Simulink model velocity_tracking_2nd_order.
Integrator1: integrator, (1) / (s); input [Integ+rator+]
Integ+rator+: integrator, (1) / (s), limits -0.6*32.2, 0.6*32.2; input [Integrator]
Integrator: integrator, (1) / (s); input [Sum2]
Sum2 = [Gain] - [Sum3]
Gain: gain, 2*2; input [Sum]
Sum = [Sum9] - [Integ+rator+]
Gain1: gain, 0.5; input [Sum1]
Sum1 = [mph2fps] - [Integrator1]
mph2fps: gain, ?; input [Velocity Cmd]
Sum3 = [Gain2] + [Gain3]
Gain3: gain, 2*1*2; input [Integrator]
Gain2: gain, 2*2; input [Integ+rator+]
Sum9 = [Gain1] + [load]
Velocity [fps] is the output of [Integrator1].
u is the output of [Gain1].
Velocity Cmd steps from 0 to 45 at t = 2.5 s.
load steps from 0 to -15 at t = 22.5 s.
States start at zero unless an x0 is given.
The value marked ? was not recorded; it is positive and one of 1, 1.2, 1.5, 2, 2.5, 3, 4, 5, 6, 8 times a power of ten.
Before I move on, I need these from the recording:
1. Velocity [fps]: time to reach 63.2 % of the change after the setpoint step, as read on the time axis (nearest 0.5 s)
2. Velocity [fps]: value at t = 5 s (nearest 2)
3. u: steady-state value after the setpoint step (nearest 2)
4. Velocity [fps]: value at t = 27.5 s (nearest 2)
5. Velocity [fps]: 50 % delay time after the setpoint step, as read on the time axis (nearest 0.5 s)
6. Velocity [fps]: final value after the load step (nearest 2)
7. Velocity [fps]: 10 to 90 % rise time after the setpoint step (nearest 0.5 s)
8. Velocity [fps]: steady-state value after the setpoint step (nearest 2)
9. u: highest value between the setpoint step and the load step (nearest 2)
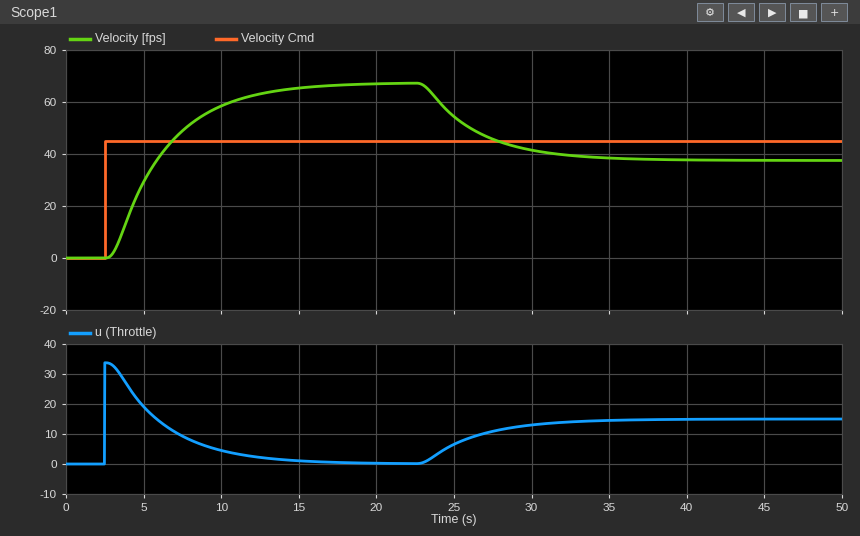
6.5 s
30
0
46
5.5 s
38
7.5 s
68
34
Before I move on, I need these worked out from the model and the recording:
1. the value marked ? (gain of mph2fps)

1.5
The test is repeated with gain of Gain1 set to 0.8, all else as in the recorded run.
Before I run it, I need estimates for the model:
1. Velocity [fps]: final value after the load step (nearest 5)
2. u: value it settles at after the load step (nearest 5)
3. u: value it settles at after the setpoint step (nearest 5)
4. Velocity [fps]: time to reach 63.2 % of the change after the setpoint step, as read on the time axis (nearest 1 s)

50
15
0
5 s
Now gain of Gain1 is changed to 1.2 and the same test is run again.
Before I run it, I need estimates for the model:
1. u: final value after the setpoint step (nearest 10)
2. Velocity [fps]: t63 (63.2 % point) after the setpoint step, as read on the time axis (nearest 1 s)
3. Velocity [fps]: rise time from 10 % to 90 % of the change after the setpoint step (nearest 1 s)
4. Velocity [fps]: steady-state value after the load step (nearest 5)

0
5 s
3 s
55
